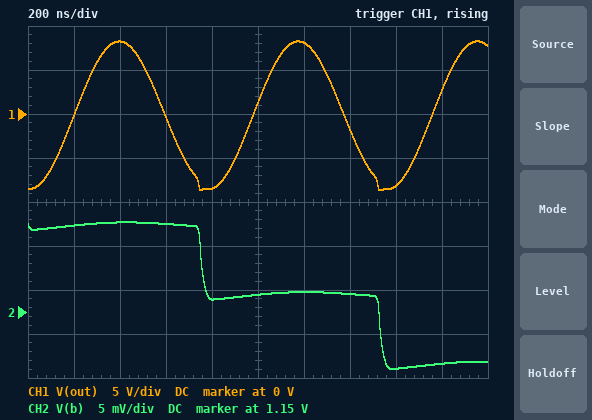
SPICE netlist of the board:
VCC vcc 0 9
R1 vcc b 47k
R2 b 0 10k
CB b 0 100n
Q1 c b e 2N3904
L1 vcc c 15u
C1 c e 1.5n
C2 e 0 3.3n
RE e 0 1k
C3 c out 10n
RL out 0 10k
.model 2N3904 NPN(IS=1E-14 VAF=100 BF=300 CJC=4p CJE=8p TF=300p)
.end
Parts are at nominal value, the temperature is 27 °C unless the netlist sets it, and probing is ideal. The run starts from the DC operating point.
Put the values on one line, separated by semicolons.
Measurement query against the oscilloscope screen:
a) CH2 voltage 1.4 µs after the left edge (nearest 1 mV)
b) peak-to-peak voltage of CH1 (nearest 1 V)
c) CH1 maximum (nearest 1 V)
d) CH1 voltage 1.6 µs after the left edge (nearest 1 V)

1.152 V; 17 V; 8 V; -8 V
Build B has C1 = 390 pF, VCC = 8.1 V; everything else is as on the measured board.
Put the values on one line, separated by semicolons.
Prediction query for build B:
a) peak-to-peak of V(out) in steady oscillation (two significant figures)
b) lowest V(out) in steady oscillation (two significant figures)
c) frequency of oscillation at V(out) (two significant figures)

15 V; -7.7 V; 2.2 MHz
